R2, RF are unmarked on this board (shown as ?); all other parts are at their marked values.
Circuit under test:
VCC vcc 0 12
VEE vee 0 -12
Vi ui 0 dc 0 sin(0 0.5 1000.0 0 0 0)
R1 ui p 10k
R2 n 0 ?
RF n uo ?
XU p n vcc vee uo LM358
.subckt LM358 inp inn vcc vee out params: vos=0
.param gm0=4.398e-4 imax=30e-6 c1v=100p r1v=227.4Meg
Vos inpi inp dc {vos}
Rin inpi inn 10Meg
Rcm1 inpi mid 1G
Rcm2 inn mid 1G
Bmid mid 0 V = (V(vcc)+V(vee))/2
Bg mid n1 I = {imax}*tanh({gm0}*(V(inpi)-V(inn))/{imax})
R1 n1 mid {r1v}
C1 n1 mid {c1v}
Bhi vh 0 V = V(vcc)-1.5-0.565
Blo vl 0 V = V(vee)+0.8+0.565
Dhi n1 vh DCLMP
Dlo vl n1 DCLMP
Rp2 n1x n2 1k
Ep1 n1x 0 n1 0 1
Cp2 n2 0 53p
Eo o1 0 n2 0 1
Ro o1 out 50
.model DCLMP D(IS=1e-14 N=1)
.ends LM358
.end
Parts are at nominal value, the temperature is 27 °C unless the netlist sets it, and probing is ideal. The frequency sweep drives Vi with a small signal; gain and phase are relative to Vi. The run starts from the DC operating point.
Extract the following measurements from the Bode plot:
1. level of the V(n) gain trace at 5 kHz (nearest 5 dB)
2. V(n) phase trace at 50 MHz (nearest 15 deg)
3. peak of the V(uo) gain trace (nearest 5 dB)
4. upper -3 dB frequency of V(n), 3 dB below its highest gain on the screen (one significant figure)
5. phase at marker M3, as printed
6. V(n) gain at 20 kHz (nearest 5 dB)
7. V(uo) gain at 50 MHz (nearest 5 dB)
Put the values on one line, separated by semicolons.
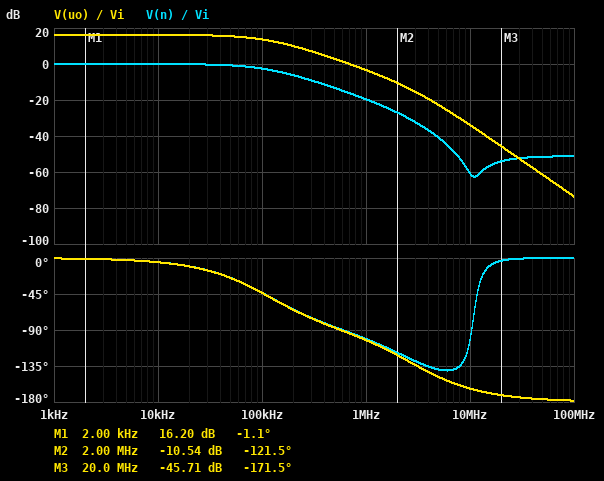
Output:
0 dB; 0 deg; 15 dB; 100 kHz; -171.5 deg; 0 dB; -60 dB
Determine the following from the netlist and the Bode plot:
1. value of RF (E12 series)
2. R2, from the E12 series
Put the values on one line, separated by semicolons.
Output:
180 kΩ; 33 kΩ
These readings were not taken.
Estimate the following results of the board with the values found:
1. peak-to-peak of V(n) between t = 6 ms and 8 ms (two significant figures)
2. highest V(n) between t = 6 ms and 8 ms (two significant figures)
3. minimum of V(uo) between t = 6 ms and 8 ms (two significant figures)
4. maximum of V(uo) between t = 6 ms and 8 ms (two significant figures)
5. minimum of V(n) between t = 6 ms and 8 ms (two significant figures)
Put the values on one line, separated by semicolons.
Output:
1.0 V; 500 mV; -3.2 V; 3.2 V; -500 mV
